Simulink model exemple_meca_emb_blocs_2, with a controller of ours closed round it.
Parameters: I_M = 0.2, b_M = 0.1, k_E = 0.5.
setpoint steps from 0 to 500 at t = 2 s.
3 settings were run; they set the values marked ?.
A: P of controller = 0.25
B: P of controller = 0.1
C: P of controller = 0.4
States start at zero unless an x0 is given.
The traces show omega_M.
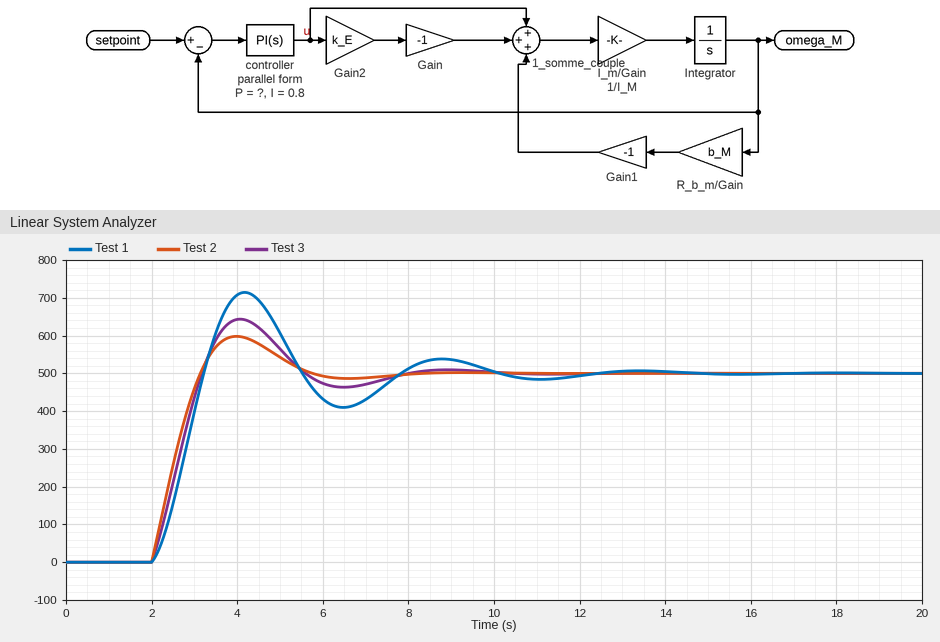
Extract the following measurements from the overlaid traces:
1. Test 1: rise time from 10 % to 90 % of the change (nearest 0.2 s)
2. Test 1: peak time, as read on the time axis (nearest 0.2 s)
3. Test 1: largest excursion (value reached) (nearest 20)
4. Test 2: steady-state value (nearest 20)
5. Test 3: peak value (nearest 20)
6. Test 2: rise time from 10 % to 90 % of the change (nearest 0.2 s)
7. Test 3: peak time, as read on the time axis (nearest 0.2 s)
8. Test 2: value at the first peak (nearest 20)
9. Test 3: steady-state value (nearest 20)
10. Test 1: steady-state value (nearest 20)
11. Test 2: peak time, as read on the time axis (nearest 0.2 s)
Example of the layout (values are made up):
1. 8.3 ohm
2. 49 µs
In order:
1. 0.8 s
2. 4.2 s
3. 720
4. 500
5. 640
6. 0.8 s
7. 4.0 s
8. 600
9. 500
10. 500
11. 4.0 s
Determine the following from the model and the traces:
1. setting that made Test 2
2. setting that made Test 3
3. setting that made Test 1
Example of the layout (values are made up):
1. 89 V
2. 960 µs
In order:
1. C
2. A
3. B
